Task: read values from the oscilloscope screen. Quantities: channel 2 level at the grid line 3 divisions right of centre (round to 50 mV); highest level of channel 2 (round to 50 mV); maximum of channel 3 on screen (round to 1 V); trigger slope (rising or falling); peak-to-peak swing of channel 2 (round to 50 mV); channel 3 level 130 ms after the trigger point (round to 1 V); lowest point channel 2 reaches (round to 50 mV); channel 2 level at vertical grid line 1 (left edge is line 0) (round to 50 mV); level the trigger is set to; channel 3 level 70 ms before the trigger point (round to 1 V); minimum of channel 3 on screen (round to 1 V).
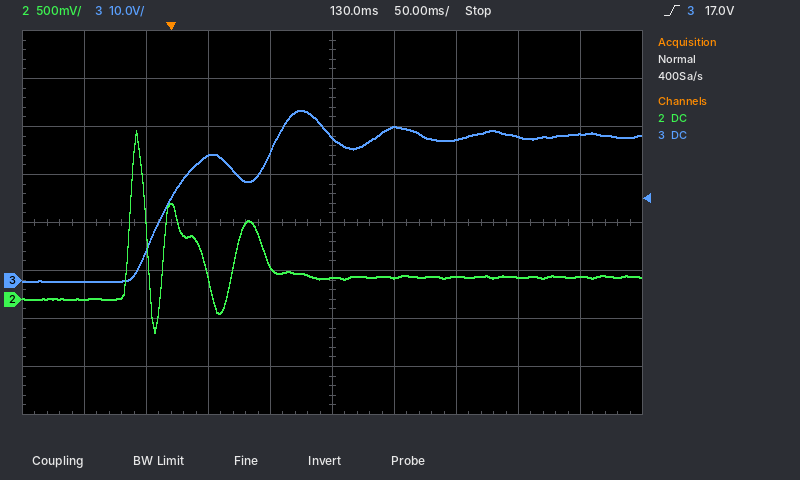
250 mV
1.75 V
35 V
rising
2.10 V
30 V
-350 mV
0 mV
17.0 V
0 V
0 V
